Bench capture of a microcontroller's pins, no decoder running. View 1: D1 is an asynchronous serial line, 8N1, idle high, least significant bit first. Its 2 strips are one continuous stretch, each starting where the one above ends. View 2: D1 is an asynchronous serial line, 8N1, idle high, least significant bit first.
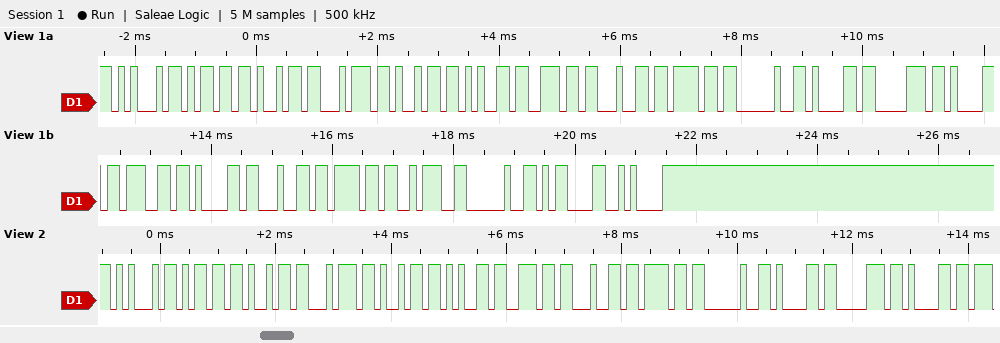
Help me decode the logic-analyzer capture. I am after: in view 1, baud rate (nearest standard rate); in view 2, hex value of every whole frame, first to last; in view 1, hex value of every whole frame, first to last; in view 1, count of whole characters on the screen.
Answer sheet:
9600 baud
45 6D 69 74 69 65 6E 64 6F 20 61 70 61
45 6D 69 74 69 65 6E 64 6F 20 61 70 61 67 61 64 6F 3A 20 0D 0A
21
